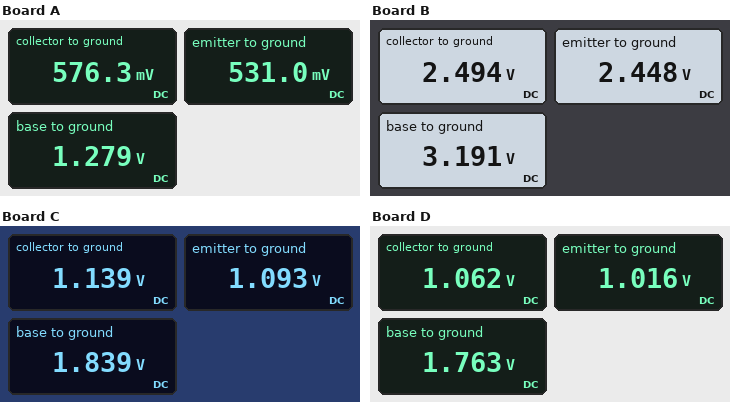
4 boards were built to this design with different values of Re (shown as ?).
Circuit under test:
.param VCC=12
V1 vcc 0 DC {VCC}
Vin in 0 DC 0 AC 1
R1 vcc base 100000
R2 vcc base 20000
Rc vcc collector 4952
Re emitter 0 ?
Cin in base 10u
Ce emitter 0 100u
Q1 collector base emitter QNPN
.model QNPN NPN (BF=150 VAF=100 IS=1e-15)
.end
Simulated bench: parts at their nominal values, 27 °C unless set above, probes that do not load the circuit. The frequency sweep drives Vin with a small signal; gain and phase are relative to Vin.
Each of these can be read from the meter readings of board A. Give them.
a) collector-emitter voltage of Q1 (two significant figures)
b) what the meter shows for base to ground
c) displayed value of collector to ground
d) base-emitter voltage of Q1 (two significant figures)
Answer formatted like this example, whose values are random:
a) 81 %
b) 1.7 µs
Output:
a) 45 mV
b) 1.279 V
c) 576.3 mV
d) 750 mV
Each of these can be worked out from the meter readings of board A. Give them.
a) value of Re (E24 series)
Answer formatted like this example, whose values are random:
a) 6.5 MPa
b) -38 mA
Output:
a) 180 Ω
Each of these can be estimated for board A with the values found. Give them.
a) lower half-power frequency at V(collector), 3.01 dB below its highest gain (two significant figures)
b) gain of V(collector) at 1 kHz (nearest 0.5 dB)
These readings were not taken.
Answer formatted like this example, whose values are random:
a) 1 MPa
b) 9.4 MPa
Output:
a) 1.2 kHz
b) 1.5 dB
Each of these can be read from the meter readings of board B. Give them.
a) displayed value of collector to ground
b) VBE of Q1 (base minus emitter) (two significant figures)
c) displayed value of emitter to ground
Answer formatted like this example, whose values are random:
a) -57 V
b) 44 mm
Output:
a) 2.494 V
b) 740 mV
c) 2.448 V
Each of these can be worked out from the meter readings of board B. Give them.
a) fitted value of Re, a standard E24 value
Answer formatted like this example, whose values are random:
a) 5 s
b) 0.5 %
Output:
a) 1 kΩ
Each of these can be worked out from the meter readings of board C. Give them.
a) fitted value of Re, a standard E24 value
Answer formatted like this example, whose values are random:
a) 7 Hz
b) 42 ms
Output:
a) 390 Ω
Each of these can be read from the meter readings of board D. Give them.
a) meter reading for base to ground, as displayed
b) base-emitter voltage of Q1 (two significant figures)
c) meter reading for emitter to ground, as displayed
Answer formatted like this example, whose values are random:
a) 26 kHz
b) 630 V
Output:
a) 1.763 V
b) 750 mV
c) 1.016 V
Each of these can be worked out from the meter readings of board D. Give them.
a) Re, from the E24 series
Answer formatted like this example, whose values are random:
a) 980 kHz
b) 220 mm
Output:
a) 360 Ω
